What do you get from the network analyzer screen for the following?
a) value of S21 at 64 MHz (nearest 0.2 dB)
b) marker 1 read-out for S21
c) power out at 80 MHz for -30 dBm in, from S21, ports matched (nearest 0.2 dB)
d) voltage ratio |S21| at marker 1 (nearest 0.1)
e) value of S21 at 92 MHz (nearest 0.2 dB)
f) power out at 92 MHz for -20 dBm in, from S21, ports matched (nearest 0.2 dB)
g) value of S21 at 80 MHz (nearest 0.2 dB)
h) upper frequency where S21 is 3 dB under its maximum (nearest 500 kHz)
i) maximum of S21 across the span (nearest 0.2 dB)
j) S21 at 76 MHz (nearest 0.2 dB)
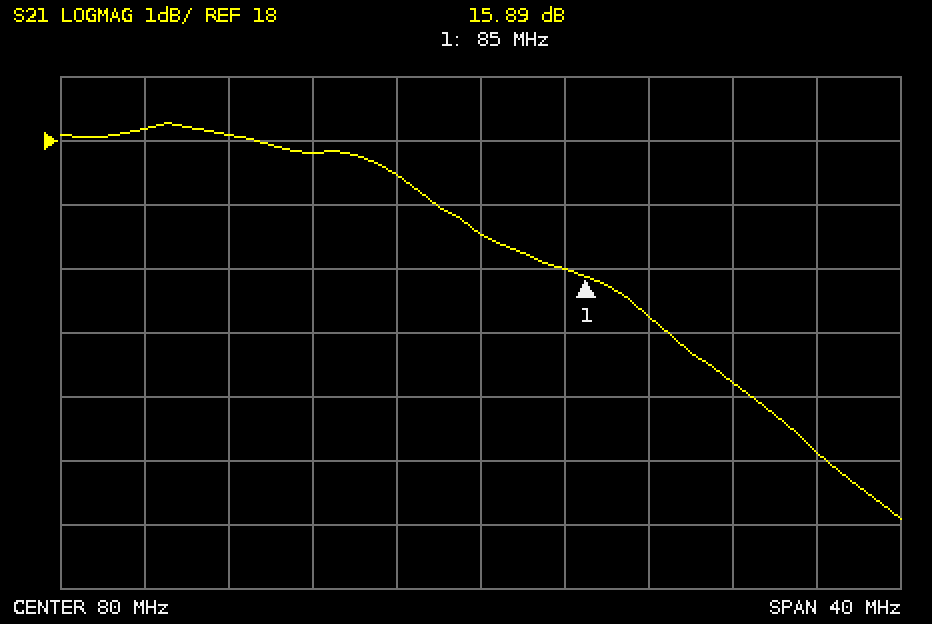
18.2 dB
15.89 dB
-13.4 dBm
6.2
14.2 dB
-5.8 dBm
16.6 dB
88.0 MHz
18.2 dB
17.4 dB
